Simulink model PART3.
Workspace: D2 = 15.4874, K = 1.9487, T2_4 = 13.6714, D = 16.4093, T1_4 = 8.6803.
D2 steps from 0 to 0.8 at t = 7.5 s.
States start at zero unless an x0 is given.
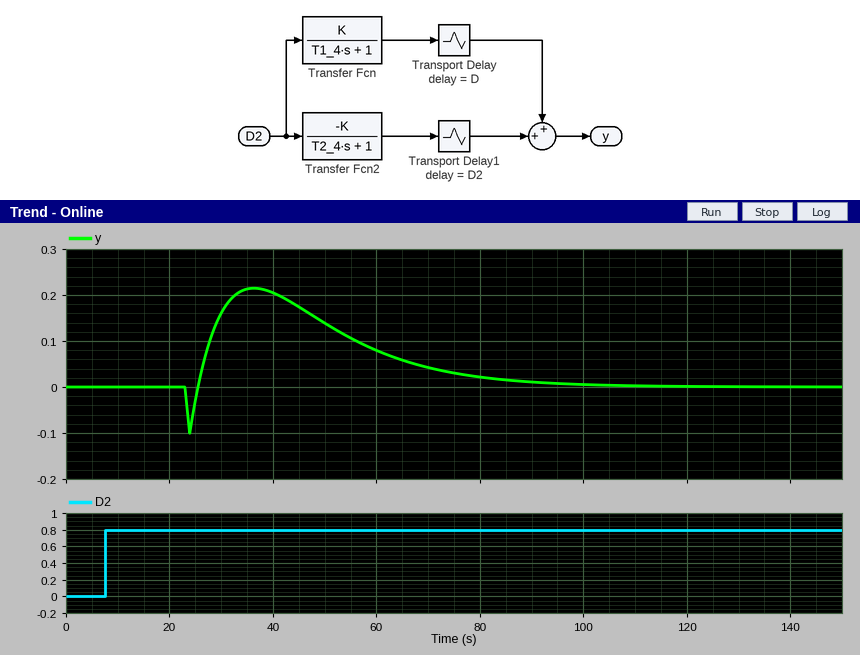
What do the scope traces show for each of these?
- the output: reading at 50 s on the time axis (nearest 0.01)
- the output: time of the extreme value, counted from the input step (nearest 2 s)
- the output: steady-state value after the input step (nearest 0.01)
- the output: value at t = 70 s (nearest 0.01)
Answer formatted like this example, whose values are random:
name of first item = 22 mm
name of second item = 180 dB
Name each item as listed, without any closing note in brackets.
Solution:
the output: reading at 50 s on the time axis = 0.14
the output: time of the extreme value, counted from the input step = 28 s
the output: steady-state value after the input step = 0.00
the output: value at t = 70 s = 0.04
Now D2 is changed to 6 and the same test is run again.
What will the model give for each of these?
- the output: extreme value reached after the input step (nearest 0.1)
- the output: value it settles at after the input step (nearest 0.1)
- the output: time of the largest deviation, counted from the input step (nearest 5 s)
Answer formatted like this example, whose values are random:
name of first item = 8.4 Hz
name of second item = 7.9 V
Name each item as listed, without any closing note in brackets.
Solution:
the output: extreme value reached after the input step = -0.8
the output: value it settles at after the input step = 0.0
the output: time of the largest deviation, counted from the input step = 15 s
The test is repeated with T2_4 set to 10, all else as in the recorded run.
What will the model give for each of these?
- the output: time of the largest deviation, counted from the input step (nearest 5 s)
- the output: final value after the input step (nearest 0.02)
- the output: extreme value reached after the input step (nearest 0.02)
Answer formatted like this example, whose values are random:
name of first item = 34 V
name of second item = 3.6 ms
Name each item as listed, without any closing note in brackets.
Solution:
the output: time of the largest deviation, counted from the input step = 15 s
the output: final value after the input step = 0.00
the output: extreme value reached after the input step = -0.14
